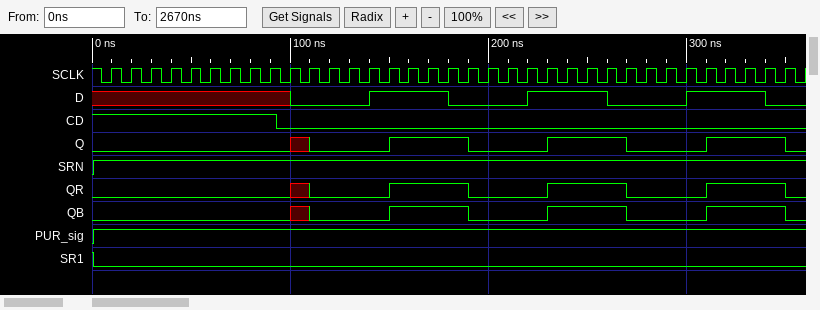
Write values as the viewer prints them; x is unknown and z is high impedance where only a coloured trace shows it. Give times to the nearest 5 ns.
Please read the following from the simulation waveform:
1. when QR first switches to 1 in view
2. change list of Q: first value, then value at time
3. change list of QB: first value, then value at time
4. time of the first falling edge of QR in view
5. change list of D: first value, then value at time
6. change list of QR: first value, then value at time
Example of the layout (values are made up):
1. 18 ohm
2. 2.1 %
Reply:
1. 150 ns
2. 0, x at 100 ns, 0 at 110 ns, 1 at 150 ns, 0 at 190 ns, 1 at 230 ns, 0 at 270 ns, 1 at 310 ns, 0 at 350 ns
3. 0, x at 100 ns, 0 at 110 ns, 1 at 150 ns, 0 at 190 ns, 1 at 230 ns, 0 at 270 ns, 1 at 310 ns, 0 at 350 ns
4. 190 ns
5. x, 0 at 100 ns, 1 at 140 ns, 0 at 180 ns, 1 at 220 ns, 0 at 260 ns, 1 at 300 ns, 0 at 340 ns
6. 0, x at 100 ns, 0 at 110 ns, 1 at 150 ns, 0 at 190 ns, 1 at 230 ns, 0 at 270 ns, 1 at 310 ns, 0 at 350 ns
